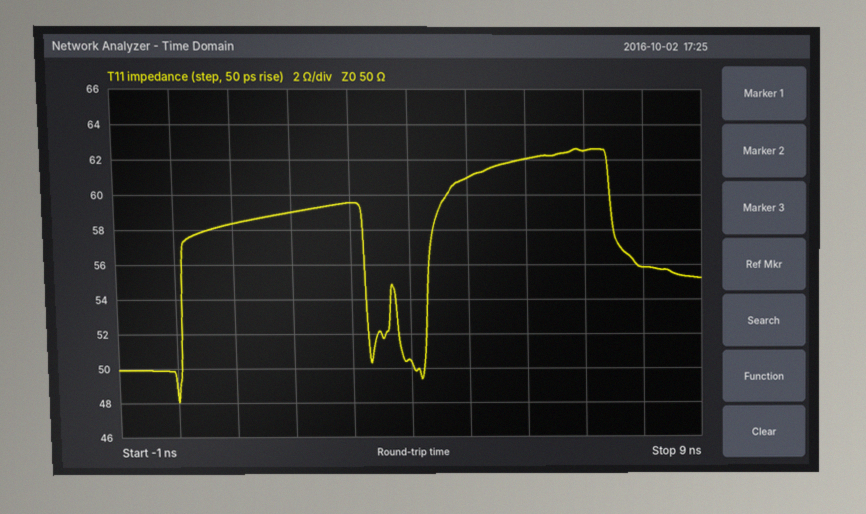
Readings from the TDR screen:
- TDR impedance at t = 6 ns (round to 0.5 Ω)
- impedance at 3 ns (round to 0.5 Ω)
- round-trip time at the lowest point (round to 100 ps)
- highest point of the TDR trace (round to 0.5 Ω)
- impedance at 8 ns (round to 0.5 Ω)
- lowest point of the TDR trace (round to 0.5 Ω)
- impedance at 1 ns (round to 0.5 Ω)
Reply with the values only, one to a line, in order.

62.0 Ω
59.5 Ω
0.0 ns
62.5 Ω
56.0 Ω
48.0 Ω
58.5 Ω
